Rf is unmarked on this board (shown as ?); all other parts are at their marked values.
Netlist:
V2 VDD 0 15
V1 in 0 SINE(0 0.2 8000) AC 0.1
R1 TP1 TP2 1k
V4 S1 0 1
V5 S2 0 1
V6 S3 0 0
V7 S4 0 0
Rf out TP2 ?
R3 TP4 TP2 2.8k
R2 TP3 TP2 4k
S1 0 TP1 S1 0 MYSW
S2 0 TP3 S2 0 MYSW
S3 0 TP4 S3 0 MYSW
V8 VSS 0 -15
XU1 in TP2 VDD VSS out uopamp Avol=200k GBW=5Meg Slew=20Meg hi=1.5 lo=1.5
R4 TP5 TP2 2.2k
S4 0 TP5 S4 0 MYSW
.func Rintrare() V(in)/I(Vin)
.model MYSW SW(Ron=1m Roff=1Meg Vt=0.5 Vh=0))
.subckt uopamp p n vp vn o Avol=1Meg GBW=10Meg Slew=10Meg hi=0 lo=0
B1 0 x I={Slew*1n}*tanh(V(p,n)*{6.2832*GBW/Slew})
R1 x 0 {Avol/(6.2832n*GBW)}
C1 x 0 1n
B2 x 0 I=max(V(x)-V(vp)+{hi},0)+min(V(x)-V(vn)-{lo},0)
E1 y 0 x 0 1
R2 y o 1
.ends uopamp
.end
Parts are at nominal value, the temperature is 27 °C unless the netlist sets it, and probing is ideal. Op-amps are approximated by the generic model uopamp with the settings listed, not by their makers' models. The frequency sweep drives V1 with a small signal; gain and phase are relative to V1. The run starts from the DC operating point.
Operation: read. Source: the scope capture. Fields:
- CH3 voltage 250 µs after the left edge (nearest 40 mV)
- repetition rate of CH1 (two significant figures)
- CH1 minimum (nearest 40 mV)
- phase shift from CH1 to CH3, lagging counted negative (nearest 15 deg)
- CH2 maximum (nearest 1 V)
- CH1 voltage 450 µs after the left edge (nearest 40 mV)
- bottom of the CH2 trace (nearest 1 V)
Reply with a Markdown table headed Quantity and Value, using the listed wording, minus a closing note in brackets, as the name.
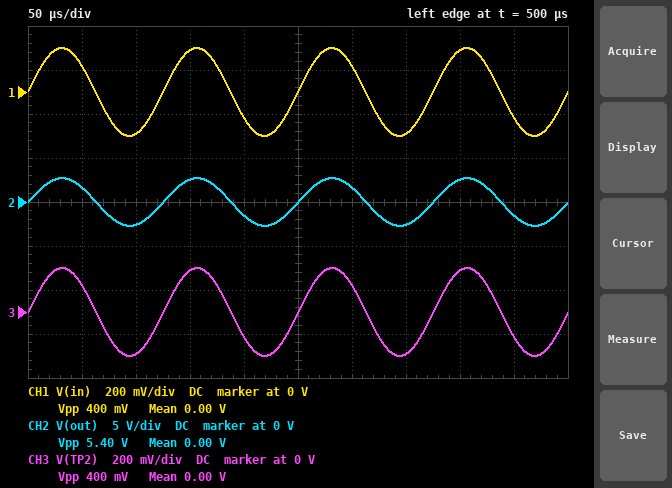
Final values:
| Quantity | Value |
|---|---|
| CH3 voltage 250 µs after the left edge | 0 V |
| repetition rate of CH1 | 8.0 kHz |
| CH1 minimum | -200 mV |
| phase shift from CH1 to CH3, lagging counted negative | 0 deg |
| CH2 maximum | 3 V |
| CH1 voltage 450 µs after the left edge | -120 mV |
| bottom of the CH2 trace | -3 V |
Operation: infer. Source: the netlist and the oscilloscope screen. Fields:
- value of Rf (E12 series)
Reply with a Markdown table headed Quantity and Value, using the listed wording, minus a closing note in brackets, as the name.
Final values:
| Quantity | Value |
|---|---|
| value of Rf | 10 kΩ |
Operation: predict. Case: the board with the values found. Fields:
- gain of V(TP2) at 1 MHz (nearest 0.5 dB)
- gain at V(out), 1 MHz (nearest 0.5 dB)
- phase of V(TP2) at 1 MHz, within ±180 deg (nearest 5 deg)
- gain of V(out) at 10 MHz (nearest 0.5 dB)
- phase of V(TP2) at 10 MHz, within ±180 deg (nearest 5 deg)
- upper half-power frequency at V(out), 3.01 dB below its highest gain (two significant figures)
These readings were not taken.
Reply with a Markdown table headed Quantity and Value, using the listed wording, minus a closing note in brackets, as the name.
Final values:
| Quantity | Value |
|---|---|
| gain of V(TP2) at 1 MHz | 0 dB |
| gain at V(out), 1 MHz | 0 dB |
| phase of V(TP2) at 1 MHz, within ±180 deg | -10 deg |
| gain of V(out) at 10 MHz | -7.0 dB |
| phase of V(TP2) at 10 MHz, within ±180 deg | -65 deg |
| upper half-power frequency at V(out), 3.01 dB below its highest gain | 4.8 MHz |
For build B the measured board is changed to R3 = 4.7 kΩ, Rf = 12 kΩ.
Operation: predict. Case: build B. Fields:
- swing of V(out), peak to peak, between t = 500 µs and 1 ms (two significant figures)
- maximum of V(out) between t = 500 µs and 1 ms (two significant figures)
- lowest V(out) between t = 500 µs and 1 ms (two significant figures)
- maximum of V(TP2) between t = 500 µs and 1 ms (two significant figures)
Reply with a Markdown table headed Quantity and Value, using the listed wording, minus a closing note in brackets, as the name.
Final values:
| Quantity | Value |
|---|---|
| swing of V(out), peak to peak, between t = 500 µs and 1 ms | 6.4 V |
| maximum of V(out) between t = 500 µs and 1 ms | 3.2 V |
| lowest V(out) between t = 500 µs and 1 ms | -3.2 V |
| maximum of V(TP2) between t = 500 µs and 1 ms | 200 mV |
